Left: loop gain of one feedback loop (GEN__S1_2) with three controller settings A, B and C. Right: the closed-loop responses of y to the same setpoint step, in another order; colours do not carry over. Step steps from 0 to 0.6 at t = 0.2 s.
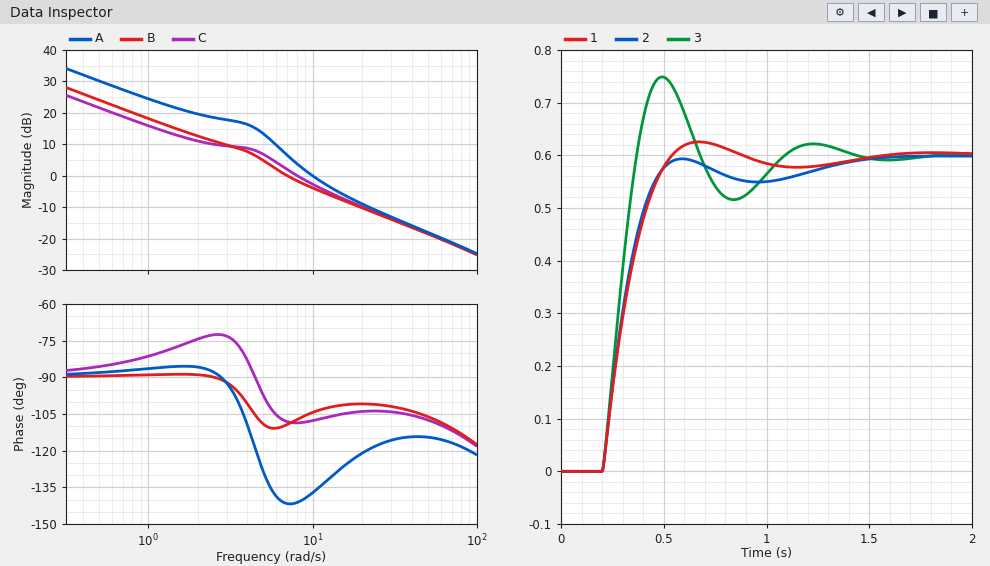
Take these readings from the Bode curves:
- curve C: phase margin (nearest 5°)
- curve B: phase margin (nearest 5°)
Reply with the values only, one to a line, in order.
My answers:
70°
70°
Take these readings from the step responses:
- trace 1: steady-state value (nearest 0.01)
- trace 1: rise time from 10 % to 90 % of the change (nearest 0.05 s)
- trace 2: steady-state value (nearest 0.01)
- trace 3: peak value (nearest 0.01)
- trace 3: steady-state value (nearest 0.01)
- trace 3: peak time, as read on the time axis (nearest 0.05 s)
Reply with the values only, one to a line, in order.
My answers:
0.60
0.25 s
0.60
0.75
0.60
0.50 s
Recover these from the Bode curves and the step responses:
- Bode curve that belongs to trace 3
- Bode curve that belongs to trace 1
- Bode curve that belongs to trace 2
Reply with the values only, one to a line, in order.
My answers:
A
B
C
